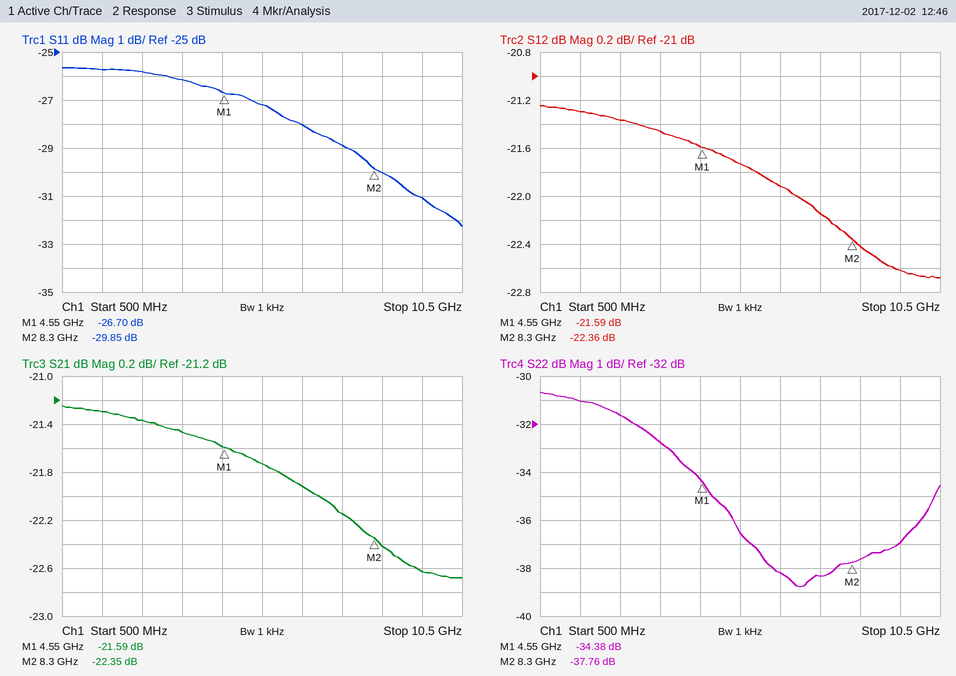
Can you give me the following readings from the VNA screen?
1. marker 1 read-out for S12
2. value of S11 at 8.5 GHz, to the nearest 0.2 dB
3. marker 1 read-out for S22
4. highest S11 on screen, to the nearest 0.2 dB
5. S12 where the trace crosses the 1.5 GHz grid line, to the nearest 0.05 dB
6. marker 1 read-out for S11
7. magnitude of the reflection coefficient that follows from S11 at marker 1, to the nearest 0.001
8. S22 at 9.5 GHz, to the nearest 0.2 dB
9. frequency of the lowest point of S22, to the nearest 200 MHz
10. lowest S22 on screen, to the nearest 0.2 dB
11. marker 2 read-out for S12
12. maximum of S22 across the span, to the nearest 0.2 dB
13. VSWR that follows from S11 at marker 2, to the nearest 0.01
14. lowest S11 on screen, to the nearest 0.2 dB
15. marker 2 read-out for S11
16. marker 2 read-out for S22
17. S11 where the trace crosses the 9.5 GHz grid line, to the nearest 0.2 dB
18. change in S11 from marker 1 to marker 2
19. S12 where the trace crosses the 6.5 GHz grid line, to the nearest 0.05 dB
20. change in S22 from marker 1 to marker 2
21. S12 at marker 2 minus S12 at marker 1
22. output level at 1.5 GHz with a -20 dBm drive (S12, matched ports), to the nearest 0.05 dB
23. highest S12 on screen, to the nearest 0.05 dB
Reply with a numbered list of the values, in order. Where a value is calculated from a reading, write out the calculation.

1. -21.59 dB
2. -30.0 dB
3. -34.38 dB
4. -25.6 dB
5. -21.30 dB
6. -26.70 dB
7. 10^(-26.7/20) ≈ 0.046
8. -37.0 dB
9. 7.0 GHz
10. -38.8 dB
11. -22.36 dB
12. -30.6 dB
13. (1 + 0.0322)/(1 − 0.0322) ≈ 1.07
14. -32.2 dB
15. -29.85 dB
16. -37.76 dB
17. -31.0 dB
18. -29.85 − (-26.7) = -3.15 dB
19. -21.90 dB
20. -37.76 − (-34.38) = -3.38 dB
21. -22.36 − (-21.59) = -0.77 dB
22. -20 dBm + (-21.30 dB) = -41.30 dBm
23. -21.25 dB
